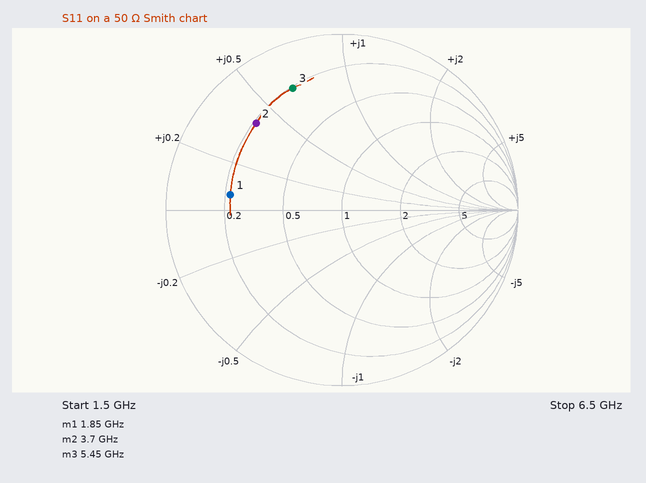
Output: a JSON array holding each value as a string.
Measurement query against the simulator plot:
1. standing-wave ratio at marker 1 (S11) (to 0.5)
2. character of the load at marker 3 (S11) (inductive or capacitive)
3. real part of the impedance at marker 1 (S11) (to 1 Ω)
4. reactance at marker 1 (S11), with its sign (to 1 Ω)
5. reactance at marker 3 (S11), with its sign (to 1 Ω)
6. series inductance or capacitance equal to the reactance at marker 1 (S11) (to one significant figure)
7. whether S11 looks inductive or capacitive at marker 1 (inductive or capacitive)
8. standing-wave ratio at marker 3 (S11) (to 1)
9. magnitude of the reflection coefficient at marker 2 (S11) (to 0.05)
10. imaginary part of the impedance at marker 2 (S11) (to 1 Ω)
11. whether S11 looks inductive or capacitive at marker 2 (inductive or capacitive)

["4.5", "inductive", "11 Ω", "+3 Ω", "+33 Ω", "300 pH", "inductive", "7", "0.70", "+20 Ω", "inductive"]
